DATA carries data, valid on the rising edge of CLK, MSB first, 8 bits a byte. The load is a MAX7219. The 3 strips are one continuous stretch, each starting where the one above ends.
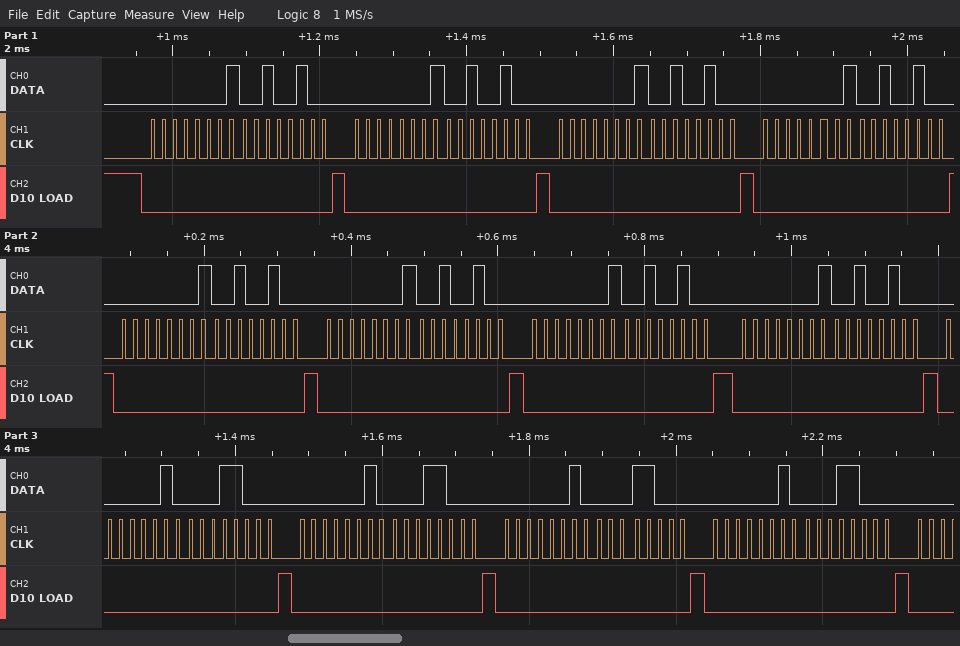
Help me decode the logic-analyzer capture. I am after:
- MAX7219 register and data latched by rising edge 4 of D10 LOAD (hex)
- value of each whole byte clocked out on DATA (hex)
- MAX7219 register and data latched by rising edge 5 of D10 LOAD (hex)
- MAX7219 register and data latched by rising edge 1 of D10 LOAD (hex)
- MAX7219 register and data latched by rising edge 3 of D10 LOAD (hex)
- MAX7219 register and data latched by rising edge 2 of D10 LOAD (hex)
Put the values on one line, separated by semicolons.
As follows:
register 0x1, data 0x24; 01 24 01 24 01 24 01 24 01 24 01 24 01 24 01 24 02 18 02 18 02 18 02 18; register 0x1, data 0x24; register 0x1, data 0x24; register 0x1, data 0x24; register 0x1, data 0x24
